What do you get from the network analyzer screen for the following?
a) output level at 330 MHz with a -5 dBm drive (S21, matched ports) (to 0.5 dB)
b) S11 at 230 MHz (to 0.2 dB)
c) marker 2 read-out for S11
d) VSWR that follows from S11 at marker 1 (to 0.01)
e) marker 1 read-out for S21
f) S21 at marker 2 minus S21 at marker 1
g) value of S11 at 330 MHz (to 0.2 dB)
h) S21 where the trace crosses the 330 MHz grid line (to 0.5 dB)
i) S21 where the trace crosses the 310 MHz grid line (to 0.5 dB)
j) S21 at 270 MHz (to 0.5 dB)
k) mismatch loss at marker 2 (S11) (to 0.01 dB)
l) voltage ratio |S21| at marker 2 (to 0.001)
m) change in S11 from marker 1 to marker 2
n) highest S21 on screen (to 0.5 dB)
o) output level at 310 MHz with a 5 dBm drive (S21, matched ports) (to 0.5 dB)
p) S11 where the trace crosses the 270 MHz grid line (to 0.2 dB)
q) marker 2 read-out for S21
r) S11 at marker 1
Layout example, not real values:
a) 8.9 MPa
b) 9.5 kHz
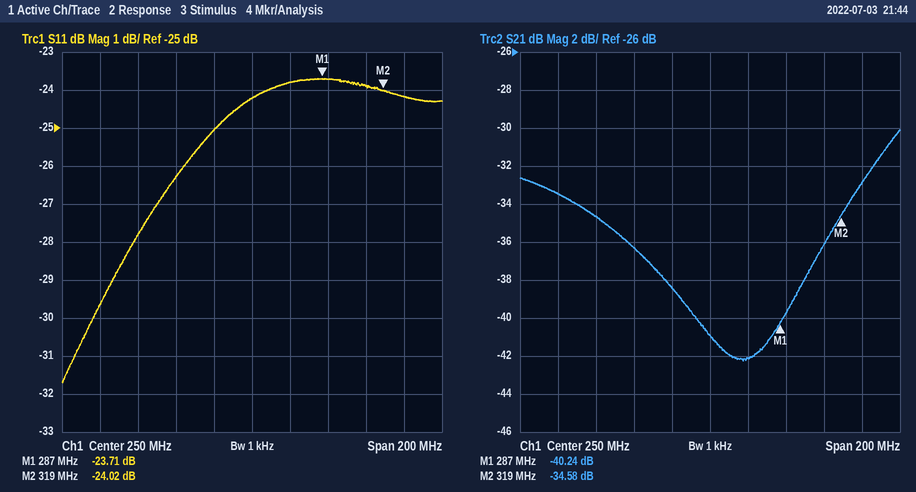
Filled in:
a) -38.0 dBm
b) -25.0 dB
c) -24.02 dB
d) 1.14
e) -40.24 dB
f) 5.66 dB
g) -24.2 dB
h) -33.0 dB
i) -36.0 dB
j) -42.0 dB
k) 0.02 dB
l) 0.019
m) -0.31 dB
n) -30.0 dB
o) -31.0 dBm
p) -23.8 dB
q) -34.58 dB
r) -23.71 dB
